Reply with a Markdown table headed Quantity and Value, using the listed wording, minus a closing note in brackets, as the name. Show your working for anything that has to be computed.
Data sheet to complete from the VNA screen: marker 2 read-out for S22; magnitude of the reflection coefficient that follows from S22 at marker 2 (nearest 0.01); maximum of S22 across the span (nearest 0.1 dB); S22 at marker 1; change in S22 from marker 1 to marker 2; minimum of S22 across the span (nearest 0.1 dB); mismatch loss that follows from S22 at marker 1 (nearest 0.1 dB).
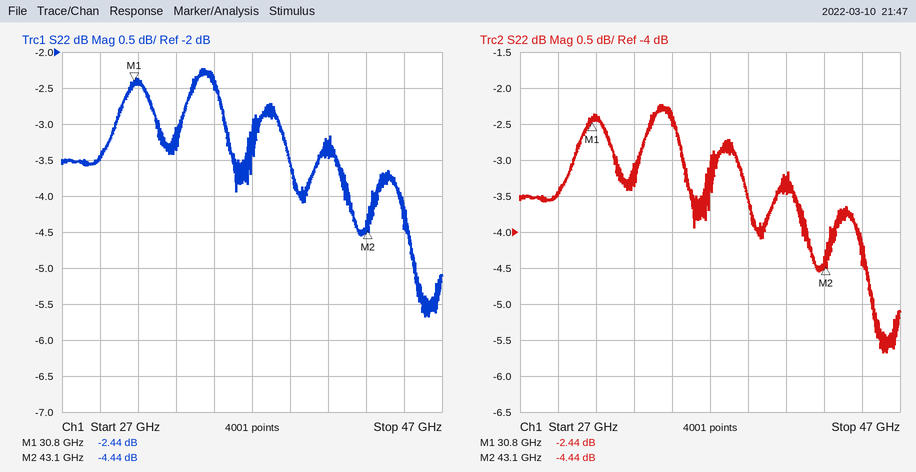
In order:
| Quantity | Value |
|---|---|
| marker 2 read-out for S22 | -4.44 dB |
| magnitude of the reflection coefficient that follows from S22 at marker 2 | 10^(-4.44/20) ≈ 0.60 |
| maximum of S22 across the span | -2.2 dB |
| S22 at marker 1 | -2.44 dB |
| change in S22 from marker 1 to marker 2 | -4.44 − (-2.44) = -2.00 dB |
| minimum of S22 across the span | -5.7 dB |
| mismatch loss that follows from S22 at marker 1 | −10 log10(1 − 10^(-2.44/10)) ≈ 3.7 dB |
